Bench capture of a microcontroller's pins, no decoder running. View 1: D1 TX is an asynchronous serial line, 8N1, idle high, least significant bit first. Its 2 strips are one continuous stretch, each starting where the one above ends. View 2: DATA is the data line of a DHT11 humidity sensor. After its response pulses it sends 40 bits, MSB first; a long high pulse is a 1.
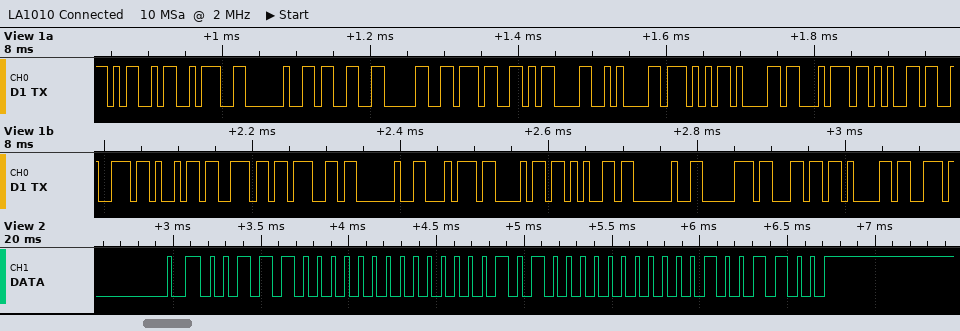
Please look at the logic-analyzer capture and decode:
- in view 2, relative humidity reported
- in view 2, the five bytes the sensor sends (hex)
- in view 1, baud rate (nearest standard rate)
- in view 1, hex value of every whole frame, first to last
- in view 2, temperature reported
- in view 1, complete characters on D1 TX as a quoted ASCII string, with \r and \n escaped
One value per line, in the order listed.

56 %
38 00 14 00 4C
115200 baud
4D 3A 20 33 30 37 0D 0A 57 61 74 65 72 69 6E 67 20 74 68 65 20 70 6C 61
20.0 °C
"M: 307\r\nWatering the pla"
